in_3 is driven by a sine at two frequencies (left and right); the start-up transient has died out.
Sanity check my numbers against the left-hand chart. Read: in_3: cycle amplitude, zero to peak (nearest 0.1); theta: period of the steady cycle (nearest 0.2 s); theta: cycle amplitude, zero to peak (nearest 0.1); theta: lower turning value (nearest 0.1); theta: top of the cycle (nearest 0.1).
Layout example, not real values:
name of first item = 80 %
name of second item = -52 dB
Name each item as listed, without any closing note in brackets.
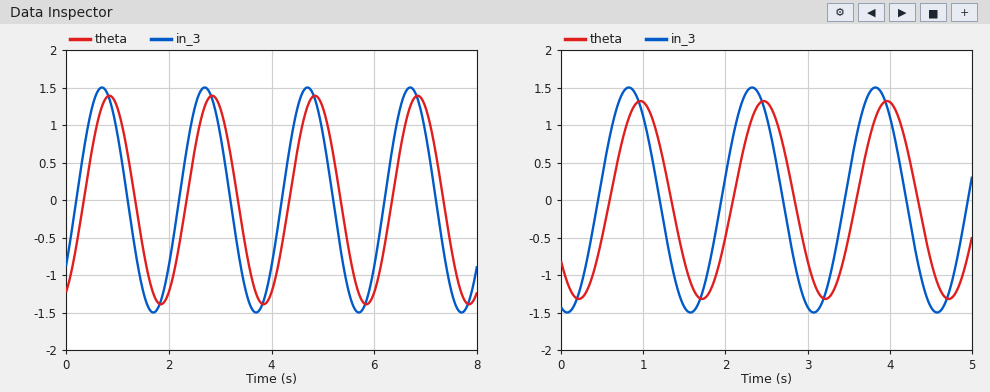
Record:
in_3: cycle amplitude, zero to peak = 1.5
theta: period of the steady cycle = 2.0 s
theta: cycle amplitude, zero to peak = 1.4
theta: lower turning value = -1.4
theta: top of the cycle = 1.4
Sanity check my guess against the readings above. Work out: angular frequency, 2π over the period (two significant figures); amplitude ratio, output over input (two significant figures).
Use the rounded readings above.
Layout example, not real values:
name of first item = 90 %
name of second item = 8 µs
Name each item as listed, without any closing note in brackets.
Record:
angular frequency, 2π over the period = 3.1 rad/s
amplitude ratio, output over input = 0.93
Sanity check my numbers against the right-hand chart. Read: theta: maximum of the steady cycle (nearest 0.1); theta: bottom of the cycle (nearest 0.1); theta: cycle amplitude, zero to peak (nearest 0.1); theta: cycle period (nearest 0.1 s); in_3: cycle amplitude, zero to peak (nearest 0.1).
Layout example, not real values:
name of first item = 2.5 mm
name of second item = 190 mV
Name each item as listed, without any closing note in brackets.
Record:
theta: maximum of the steady cycle = 1.3
theta: bottom of the cycle = -1.3
theta: cycle amplitude, zero to peak = 1.3
theta: cycle period = 1.5 s
in_3: cycle amplitude, zero to peak = 1.5
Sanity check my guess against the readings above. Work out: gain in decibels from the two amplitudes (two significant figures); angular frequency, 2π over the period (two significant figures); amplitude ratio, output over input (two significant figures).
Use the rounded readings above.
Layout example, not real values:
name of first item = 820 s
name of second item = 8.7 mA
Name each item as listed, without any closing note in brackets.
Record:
gain in decibels from the two amplitudes = -1.2 dB
angular frequency, 2π over the period = 4.2 rad/s
amplitude ratio, output over input = 0.87
